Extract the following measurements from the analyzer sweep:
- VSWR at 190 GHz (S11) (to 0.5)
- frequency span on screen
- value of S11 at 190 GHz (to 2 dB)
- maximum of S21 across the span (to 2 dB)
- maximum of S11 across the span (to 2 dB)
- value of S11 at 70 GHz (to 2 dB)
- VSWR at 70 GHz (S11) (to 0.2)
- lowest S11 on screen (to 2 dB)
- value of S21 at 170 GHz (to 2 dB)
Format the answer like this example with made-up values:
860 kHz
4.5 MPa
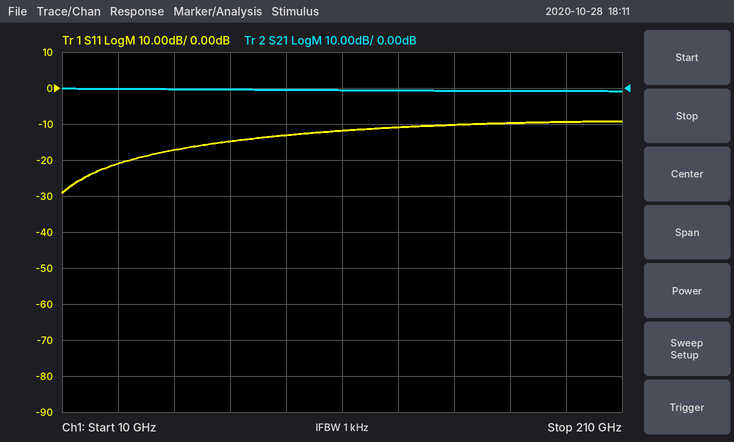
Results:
2.0
200 GHz
-10 dB
0 dB
-10 dB
-14 dB
1.4
-30 dB
0 dB
